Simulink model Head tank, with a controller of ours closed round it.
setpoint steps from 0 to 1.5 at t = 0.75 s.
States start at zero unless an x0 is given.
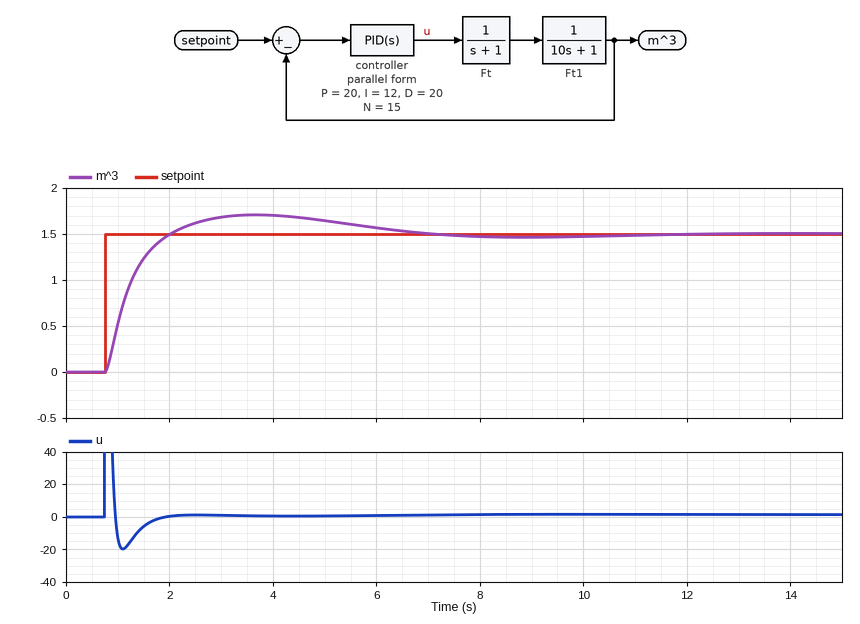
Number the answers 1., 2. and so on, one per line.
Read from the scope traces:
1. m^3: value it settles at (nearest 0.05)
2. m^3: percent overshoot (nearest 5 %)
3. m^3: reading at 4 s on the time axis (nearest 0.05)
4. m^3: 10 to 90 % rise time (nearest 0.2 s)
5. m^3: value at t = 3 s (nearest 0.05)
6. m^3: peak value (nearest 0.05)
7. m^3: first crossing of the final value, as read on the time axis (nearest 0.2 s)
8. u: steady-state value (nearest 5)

1. 1.50
2. 15 %
3. 1.70
4. 0.8 s
5. 1.70
6. 1.70
7. 2.0 s
8. 0
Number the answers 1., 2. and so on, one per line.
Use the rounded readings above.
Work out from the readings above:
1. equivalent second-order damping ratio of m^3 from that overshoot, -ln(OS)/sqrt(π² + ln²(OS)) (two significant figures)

1. 0.52
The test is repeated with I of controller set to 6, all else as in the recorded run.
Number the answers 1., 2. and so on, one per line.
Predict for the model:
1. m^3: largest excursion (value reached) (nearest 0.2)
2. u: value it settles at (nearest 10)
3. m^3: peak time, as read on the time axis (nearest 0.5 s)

1. 1.6
2. 0
3. 4.5 s
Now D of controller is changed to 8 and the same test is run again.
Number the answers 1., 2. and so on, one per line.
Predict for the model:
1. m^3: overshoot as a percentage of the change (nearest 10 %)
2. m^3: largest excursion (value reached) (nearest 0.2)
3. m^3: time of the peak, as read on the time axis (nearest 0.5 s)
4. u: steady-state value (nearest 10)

1. 30 %
2. 2.0
3. 3.0 s
4. 0
